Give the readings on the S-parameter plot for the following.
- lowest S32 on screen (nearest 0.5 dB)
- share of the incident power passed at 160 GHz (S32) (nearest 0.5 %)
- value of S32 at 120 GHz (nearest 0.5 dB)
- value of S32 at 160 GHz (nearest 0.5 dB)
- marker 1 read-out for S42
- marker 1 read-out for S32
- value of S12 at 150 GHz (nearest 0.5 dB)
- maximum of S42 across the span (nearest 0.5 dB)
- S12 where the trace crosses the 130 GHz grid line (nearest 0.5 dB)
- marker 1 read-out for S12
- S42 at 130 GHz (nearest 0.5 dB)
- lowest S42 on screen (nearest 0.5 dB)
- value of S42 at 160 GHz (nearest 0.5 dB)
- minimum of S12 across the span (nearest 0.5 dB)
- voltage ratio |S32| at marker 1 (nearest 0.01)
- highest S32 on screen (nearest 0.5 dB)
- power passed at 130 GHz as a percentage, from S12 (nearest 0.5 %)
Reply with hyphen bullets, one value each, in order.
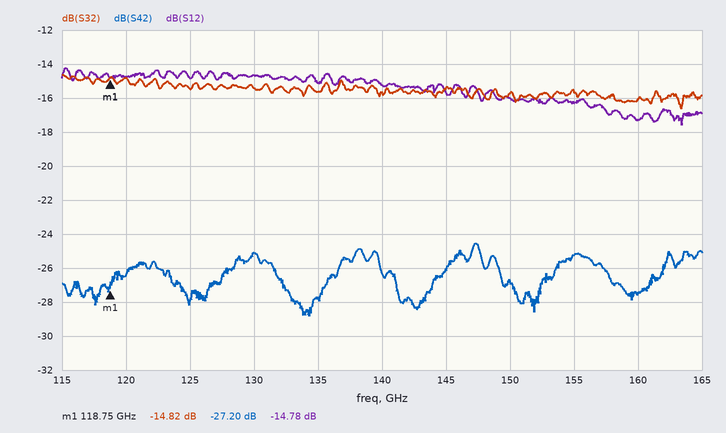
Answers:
- -16.5 dB
- 2.5 %
- -15.0 dB
- -16.0 dB
- -27.20 dB
- -14.82 dB
- -16.0 dB
- -24.5 dB
- -14.5 dB
- -14.78 dB
- -25.0 dB
- -29.0 dB
- -27.5 dB
- -17.5 dB
- 0.18
- -14.5 dB
- 3.5 %
